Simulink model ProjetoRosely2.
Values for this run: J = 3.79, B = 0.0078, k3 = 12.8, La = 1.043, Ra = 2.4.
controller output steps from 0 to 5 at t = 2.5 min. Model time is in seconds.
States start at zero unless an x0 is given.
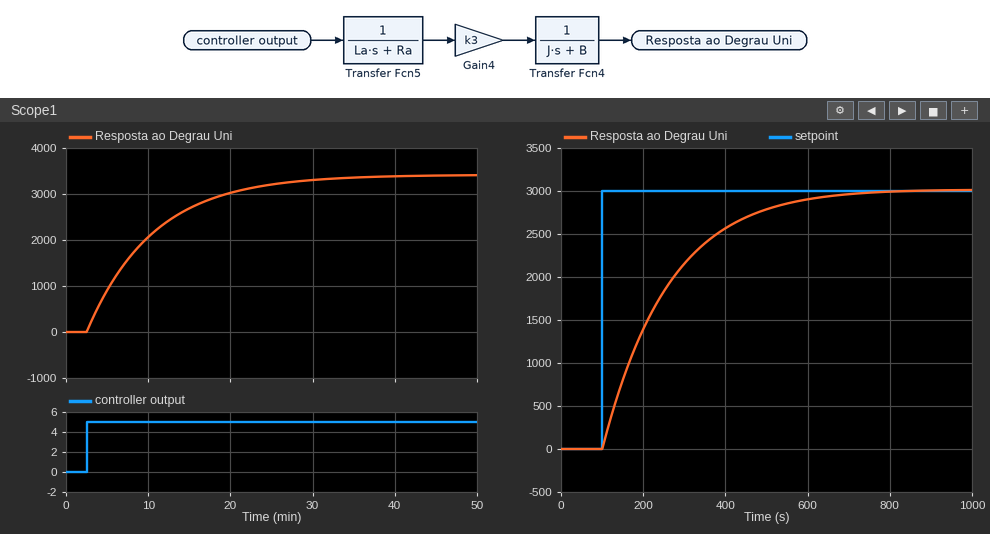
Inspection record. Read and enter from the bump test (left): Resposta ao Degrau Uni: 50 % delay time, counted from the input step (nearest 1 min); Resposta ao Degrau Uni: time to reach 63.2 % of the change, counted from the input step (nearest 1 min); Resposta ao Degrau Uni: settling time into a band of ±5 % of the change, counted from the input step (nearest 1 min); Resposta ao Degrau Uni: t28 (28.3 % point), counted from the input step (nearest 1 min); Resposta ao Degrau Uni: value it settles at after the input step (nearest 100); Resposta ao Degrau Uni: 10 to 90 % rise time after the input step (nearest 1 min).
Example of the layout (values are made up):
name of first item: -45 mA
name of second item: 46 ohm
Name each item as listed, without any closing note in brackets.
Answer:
Resposta ao Degrau Uni: 50 % delay time, counted from the input step: 6 min
Resposta ao Degrau Uni: time to reach 63.2 % of the change, counted from the input step: 8 min
Resposta ao Degrau Uni: settling time into a band of ±5 % of the change, counted from the input step: 24 min
Resposta ao Degrau Uni: t28 (28.3 % point), counted from the input step: 3 min
Resposta ao Degrau Uni: value it settles at after the input step: 3400
Resposta ao Degrau Uni: 10 to 90 % rise time after the input step: 18 min
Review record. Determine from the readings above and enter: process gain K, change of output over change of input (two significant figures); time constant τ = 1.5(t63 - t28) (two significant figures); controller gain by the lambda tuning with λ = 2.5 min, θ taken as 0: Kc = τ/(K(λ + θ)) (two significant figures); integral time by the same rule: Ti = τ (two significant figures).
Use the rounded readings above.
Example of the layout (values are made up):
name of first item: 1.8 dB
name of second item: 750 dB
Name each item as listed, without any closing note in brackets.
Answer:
process gain K, change of output over change of input: 680
time constant τ = 1.5(t63 - t28): 7.5 min
controller gain by the lambda tuning with λ = 2.5 min, θ taken as 0: Kc = τ/(K(λ + θ)): 0.0044
integral time by the same rule: Ti = τ: 7.5 min
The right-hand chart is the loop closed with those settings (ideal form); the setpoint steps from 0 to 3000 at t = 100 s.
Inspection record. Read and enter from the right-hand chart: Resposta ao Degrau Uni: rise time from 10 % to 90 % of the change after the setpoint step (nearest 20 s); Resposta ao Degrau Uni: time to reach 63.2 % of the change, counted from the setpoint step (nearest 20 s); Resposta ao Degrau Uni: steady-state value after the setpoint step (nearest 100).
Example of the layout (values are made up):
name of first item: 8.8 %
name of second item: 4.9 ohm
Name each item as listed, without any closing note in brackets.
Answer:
Resposta ao Degrau Uni: rise time from 10 % to 90 % of the change after the setpoint step: 340 s
Resposta ao Degrau Uni: time to reach 63.2 % of the change, counted from the setpoint step: 160 s
Resposta ao Degrau Uni: steady-state value after the setpoint step: 3000
